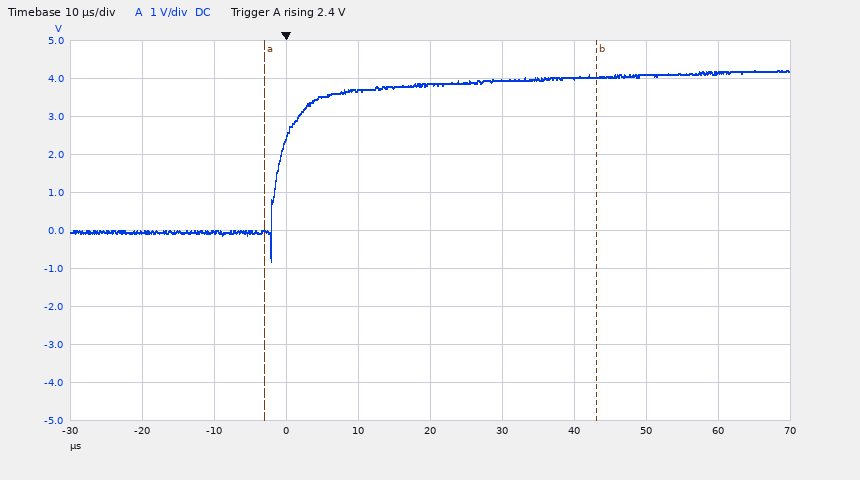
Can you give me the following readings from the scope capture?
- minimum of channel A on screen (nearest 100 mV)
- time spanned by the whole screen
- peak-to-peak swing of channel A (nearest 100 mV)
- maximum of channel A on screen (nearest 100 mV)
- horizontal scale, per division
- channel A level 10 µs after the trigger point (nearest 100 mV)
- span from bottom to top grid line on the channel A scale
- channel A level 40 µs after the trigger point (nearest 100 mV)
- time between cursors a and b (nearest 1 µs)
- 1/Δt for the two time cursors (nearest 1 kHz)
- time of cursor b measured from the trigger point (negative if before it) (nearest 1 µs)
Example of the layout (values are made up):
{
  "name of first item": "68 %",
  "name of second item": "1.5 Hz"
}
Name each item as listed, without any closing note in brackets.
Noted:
{
  "minimum of channel A on screen": "-800 mV",
  "time spanned by the whole screen": "100 µs",
  "peak-to-peak swing of channel A": "5.0 V",
  "maximum of channel A on screen": "4.2 V",
  "horizontal scale, per division": "10 µs",
  "channel A level 10 µs after the trigger point": "3.7 V",
  "span from bottom to top grid line on the channel A scale": "10 V",
  "channel A level 40 µs after the trigger point": "4.0 V",
  "time between cursors a and b": "46 µs",
  "1/Δt for the two time cursors": "22 kHz",
  "time of cursor b measured from the trigger point (negative if before it)": "+43 µs"
}
